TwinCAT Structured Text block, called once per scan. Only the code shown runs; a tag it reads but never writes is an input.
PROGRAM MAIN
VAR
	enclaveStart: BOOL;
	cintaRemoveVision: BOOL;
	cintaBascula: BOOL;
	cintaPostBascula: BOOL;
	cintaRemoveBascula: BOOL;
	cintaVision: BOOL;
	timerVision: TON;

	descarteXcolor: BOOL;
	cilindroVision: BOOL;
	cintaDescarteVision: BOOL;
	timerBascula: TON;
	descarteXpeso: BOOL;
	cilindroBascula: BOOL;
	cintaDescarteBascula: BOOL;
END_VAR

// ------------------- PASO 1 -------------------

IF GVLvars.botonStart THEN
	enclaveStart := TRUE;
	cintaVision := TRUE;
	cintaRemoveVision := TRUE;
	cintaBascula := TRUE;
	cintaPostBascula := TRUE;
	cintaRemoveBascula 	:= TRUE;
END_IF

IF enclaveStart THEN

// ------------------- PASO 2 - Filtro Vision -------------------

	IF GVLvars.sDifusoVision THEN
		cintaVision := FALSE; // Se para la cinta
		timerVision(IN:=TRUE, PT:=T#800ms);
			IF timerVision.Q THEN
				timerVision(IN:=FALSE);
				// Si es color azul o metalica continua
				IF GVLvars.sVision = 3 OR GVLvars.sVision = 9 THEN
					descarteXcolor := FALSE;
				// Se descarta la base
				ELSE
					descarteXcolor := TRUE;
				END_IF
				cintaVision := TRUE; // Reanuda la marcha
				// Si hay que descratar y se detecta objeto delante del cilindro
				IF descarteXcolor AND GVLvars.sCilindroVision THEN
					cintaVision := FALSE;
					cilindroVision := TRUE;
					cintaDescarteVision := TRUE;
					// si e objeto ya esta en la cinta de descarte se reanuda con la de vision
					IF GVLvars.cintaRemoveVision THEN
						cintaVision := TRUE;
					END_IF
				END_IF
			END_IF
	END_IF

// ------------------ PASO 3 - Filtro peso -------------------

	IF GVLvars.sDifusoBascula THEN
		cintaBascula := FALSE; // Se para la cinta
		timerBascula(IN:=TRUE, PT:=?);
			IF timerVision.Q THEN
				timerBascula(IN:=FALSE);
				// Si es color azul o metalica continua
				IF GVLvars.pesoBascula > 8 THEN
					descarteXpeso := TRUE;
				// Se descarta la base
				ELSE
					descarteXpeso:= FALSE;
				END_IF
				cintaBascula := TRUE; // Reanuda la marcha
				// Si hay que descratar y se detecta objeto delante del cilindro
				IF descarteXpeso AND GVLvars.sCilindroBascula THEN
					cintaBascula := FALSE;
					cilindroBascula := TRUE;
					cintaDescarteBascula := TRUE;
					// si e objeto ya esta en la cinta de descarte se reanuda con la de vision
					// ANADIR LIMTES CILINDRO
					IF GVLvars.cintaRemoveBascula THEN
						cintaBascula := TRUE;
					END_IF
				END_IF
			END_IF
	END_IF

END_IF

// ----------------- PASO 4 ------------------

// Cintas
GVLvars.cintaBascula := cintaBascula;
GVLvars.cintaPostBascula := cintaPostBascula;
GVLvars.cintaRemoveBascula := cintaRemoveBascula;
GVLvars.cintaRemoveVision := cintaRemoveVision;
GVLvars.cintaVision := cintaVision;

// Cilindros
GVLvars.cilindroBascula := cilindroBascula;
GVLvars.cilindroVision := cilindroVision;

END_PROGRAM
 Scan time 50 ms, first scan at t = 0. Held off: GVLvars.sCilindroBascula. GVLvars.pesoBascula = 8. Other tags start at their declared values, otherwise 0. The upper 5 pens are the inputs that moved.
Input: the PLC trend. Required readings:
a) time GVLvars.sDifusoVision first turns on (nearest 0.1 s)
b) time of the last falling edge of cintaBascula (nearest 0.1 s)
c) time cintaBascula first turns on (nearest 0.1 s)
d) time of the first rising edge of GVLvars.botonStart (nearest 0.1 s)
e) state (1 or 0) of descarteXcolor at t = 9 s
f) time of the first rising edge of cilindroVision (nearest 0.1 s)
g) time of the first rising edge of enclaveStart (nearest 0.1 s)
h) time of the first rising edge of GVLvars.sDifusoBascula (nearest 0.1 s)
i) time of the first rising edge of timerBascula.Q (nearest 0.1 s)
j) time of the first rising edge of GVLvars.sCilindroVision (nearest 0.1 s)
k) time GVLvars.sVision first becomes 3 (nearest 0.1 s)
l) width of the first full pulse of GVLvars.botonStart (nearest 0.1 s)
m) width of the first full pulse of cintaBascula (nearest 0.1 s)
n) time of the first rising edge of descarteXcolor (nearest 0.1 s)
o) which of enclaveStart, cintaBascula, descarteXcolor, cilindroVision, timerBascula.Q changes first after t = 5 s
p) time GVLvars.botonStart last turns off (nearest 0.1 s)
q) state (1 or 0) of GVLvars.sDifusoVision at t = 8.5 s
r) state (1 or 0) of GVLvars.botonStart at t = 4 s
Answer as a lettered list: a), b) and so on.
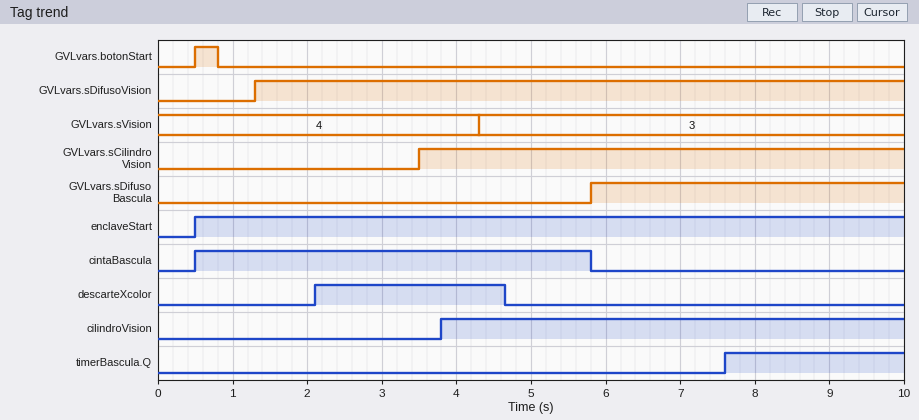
a) 1.3 s
b) 5.8 s
c) 0.5 s
d) 0.5 s
e) 0
f) 3.8 s
g) 0.5 s
h) 5.8 s
i) 7.6 s
j) 3.5 s
k) 4.3 s
l) 0.3 s
m) 5.3 s
n) 2.1 s
o) cintaBascula
p) 0.8 s
q) 1
r) 0
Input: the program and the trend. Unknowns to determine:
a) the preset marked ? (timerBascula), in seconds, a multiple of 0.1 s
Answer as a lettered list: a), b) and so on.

a) 1.8 s
